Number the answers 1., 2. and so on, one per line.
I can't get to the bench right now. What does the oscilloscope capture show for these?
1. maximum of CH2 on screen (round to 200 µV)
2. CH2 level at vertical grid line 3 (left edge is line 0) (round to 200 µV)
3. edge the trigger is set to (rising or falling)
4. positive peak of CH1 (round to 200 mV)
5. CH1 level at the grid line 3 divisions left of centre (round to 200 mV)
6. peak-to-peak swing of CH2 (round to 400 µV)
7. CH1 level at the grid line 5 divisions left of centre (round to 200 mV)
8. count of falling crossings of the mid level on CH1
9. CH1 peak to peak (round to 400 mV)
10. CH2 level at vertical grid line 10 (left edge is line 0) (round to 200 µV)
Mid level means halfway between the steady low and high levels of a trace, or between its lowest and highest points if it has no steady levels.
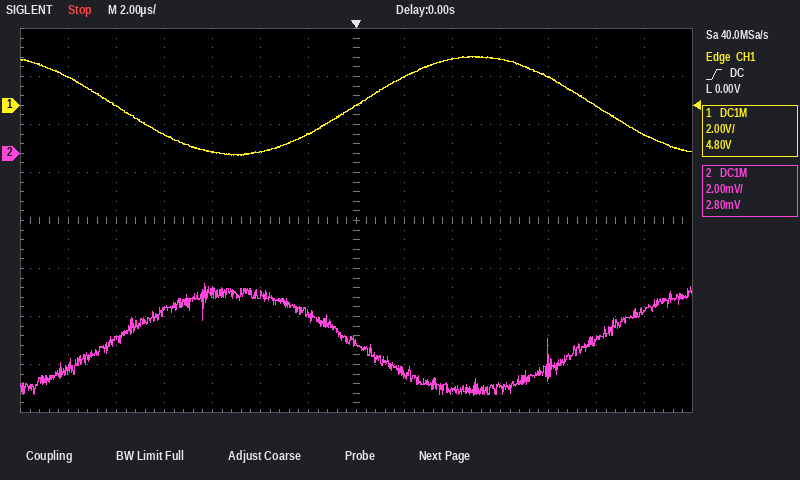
1. -5.4 mV
2. -6.6 mV
3. rising
4. 2.0 V
5. -2.0 V
6. 4.8 mV
7. 0.0 V
8. 2
9. 4.0 V
10. -9.6 mV
